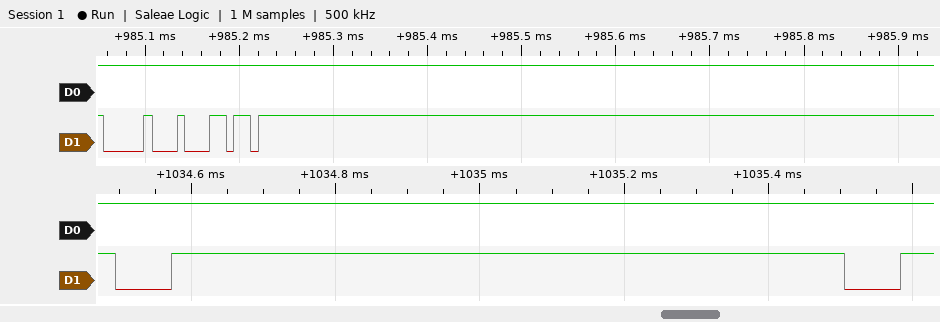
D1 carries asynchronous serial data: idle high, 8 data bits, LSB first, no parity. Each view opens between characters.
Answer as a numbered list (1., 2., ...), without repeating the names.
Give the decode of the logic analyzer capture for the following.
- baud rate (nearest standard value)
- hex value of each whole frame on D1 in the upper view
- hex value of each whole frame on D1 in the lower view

1. 115200 baud
2. 10, 6C
3. 00, 00
